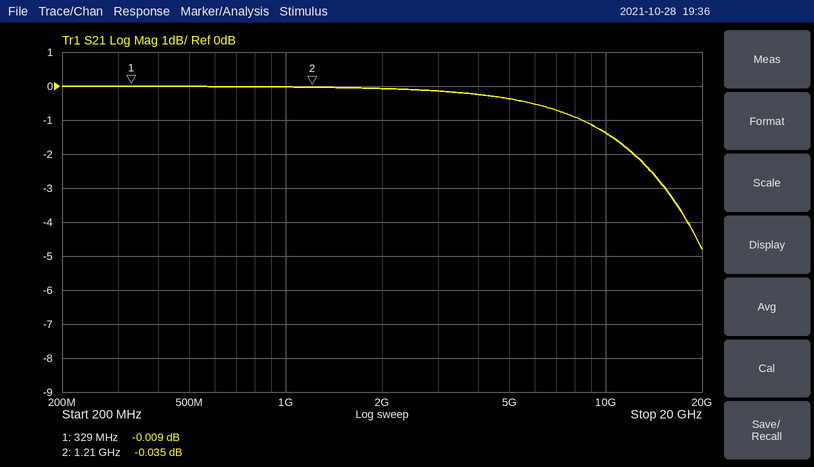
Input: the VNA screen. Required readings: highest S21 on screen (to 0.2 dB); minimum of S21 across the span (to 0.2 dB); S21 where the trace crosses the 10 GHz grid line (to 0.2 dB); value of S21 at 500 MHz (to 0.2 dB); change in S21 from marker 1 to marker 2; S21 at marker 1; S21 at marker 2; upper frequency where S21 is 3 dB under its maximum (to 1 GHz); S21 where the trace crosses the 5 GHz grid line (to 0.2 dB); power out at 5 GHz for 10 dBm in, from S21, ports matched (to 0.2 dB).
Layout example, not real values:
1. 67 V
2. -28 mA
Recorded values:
1. 0.0 dB
2. -4.8 dB
3. -1.4 dB
4. 0.0 dB
5. -0.026 dB
6. -0.009 dB
7. -0.035 dB
8. 15 GHz
9. -0.4 dB
10. 9.6 dBm
